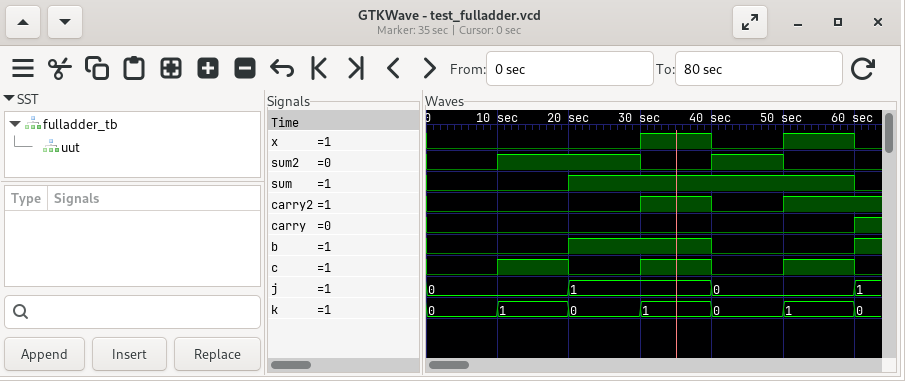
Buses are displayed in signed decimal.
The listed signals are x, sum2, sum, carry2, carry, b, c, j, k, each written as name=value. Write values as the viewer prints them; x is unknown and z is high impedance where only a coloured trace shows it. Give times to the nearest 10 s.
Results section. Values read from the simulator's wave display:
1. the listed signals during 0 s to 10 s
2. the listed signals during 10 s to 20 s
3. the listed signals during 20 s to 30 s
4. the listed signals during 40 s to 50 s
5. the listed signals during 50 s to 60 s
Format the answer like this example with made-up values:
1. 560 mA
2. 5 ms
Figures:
1. x=0, sum2=0, sum=0, carry2=0, carry=0, b=0, c=0, j=0, k=0
2. x=0, sum2=1, sum=0, carry2=0, carry=0, b=0, c=1, j=0, k=1
3. x=0, sum2=1, sum=1, carry2=0, carry=0, b=1, c=0, j=1, k=0
4. x=0, sum2=1, sum=1, carry2=0, carry=0, b=0, c=0, j=0, k=0
5. x=1, sum2=0, sum=1, carry2=1, carry=0, b=0, c=1, j=0, k=1
